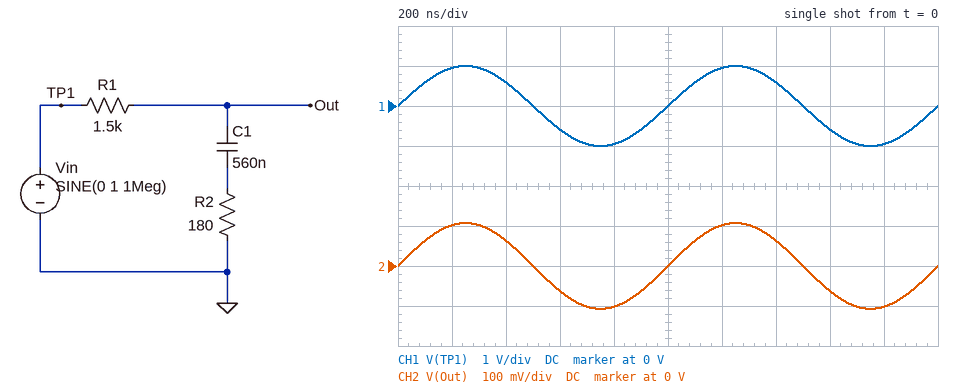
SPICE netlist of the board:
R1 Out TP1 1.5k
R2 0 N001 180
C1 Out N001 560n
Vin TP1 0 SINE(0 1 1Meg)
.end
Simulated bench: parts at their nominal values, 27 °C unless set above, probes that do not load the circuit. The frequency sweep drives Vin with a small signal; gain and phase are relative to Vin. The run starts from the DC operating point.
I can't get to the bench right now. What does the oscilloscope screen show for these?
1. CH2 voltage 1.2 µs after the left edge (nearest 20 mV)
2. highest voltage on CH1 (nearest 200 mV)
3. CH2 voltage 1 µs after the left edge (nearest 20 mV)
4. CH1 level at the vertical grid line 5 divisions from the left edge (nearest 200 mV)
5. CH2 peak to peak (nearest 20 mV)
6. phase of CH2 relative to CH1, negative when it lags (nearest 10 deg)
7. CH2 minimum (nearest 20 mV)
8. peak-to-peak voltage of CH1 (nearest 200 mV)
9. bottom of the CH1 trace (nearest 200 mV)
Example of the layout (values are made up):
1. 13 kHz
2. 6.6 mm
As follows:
1. 100 mV
2. 1.0 V
3. 0 V
4. 0 V
5. 220 mV
6. 0 deg
7. -100 mV
8. 2.0 V
9. -1.0 V
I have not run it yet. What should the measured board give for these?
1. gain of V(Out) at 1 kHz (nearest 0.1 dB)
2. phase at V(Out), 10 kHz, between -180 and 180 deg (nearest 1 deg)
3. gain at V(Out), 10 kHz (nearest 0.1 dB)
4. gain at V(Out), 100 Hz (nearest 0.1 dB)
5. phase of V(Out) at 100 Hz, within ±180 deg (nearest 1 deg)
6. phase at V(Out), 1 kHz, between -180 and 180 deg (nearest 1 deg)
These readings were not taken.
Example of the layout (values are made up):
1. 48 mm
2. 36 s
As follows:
1. -14.1 dB
2. -8 deg
3. -19.3 dB
4. -1.3 dB
5. -27 deg
6. -48 deg
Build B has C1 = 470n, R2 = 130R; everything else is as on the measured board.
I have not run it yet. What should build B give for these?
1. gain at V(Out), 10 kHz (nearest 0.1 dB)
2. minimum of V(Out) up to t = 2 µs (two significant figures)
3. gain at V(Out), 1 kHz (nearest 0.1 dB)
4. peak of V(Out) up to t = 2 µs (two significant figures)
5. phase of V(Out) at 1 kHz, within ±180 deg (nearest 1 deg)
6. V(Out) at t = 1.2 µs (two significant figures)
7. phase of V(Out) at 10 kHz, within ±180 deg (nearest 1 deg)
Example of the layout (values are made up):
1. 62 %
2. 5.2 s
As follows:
1. -21.7 dB
2. -80 mV
3. -13.2 dB
4. 80 mV
5. -57 deg
6. 76 mV
7. -13 deg
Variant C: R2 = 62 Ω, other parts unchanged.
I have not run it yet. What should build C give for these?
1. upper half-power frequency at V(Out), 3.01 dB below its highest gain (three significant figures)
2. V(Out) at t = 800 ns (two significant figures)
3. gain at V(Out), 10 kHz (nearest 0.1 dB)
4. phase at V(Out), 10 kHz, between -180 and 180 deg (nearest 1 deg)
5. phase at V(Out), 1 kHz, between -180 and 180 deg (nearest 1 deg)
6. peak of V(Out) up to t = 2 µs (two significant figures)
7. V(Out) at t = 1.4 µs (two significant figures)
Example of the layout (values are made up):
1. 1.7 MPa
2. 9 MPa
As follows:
1. 182 Hz
2. -38 mV
3. -27.2 dB
4. -24 deg
5. -67 deg
6. 40 mV
7. 24 mV
